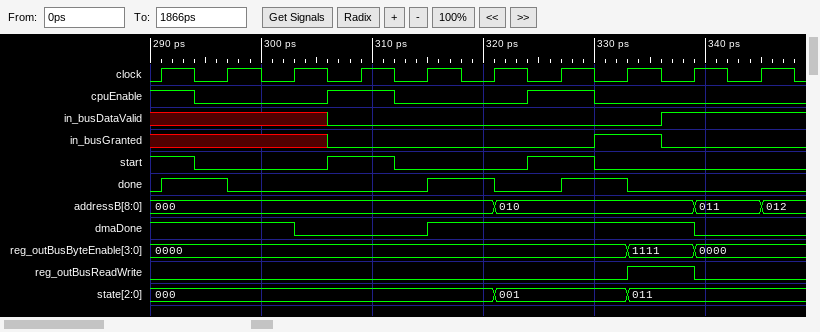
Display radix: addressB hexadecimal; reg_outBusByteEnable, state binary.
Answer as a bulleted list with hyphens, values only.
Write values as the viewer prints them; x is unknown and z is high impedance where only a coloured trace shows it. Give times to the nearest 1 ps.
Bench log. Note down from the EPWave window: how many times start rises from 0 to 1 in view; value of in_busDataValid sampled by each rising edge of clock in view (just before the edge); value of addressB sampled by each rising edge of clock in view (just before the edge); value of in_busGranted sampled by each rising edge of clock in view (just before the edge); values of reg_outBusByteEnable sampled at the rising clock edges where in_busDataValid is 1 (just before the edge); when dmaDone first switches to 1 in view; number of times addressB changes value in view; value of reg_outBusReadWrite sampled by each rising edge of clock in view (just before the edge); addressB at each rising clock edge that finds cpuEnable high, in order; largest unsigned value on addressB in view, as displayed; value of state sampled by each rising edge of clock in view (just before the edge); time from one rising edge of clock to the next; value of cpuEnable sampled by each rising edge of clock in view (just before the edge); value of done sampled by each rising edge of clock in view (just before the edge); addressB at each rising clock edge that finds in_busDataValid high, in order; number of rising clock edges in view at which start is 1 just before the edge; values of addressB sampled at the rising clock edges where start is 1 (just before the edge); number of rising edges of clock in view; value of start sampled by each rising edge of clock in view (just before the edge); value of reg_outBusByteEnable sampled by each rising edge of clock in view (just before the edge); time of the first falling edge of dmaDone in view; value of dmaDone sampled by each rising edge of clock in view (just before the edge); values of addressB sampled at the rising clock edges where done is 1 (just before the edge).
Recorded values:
- 2
- x x x 0 0 0 0 0 1 1
- 000, 000, 000, 000, 000, 000, 010, 010, 010, 011
- x x x 0 0 0 0 1 0 0
- 1111, 0000
- 315 ps
- 3
- 0 0 0 0 0 0 0 0 1 0
- 000, 000, 010
- 012
- 000, 000, 000, 000, 000, 000, 001, 001, 011, 011
- 6 ps
- 1 0 0 1 0 0 1 0 0 0
- 0 1 0 0 0 1 0 1 0 0
- 010, 011
- 3
- 000, 000, 010
- 10
- 1 0 0 1 0 0 1 0 0 0
- 0000, 0000, 0000, 0000, 0000, 0000, 0000, 0000, 1111, 0000
- 303 ps
- 1 1 1 0 0 1 1 1 1 0
- 000, 000, 010
